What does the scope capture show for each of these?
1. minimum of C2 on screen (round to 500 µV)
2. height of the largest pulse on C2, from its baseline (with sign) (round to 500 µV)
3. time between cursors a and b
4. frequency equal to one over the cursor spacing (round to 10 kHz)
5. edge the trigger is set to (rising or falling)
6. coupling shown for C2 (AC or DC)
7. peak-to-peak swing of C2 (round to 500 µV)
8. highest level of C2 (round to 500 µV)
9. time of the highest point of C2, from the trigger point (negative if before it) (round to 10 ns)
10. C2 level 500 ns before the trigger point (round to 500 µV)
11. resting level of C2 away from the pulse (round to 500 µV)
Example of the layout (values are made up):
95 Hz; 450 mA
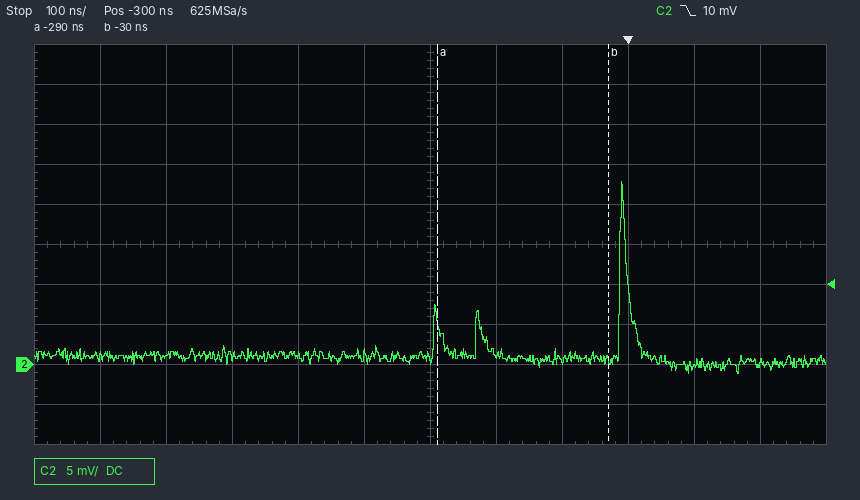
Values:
-1.0 mV; +22.0 mV; 260 ns; 3.85 MHz; falling; DC; 24.0 mV; 23.0 mV; -10 ns; 1.0 mV; 1.0 mV
